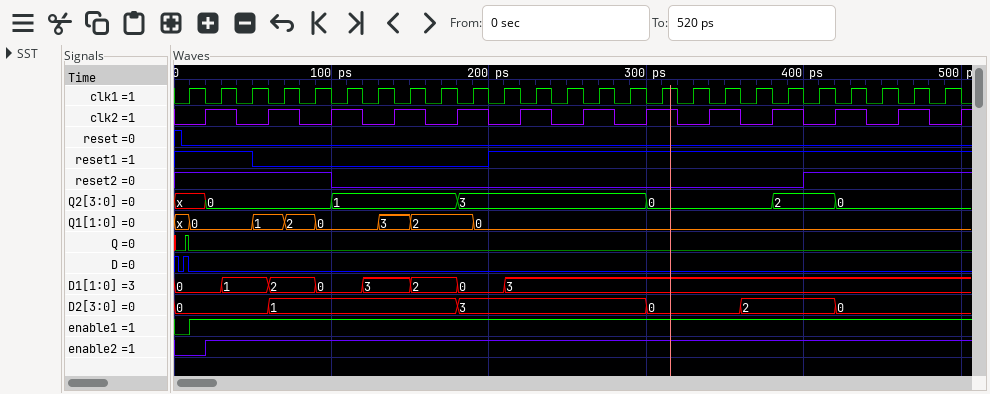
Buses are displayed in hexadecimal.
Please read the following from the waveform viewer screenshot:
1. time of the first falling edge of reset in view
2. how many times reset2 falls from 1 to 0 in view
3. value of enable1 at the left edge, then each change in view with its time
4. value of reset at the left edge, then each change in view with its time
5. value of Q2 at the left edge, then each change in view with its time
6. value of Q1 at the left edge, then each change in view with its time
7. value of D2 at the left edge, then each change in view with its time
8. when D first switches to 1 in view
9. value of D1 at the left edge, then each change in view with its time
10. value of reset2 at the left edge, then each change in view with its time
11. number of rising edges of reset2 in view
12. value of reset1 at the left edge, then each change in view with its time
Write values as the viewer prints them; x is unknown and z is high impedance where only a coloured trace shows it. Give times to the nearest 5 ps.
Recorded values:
5 ps
1
0, 1 at 10 ps
1, 0 at 5 ps
x, 0 at 20 ps, 1 at 100 ps, 3 at 180 ps, 0 at 300 ps, 2 at 380 ps, 0 at 420 ps
x, 0 at 10 ps, 1 at 50 ps, 2 at 70 ps, 0 at 90 ps, 3 at 130 ps, 2 at 150 ps, 0 at 190 ps
0, 1 at 60 ps, 3 at 180 ps, 0 at 300 ps, 2 at 360 ps, 0 at 420 ps
5 ps
0, 1 at 30 ps, 2 at 60 ps, 0 at 90 ps, 3 at 120 ps, 2 at 150 ps, 0 at 180 ps, 3 at 210 ps
1, 0 at 100 ps, 1 at 400 ps
1
1, 0 at 50 ps, 1 at 200 ps
